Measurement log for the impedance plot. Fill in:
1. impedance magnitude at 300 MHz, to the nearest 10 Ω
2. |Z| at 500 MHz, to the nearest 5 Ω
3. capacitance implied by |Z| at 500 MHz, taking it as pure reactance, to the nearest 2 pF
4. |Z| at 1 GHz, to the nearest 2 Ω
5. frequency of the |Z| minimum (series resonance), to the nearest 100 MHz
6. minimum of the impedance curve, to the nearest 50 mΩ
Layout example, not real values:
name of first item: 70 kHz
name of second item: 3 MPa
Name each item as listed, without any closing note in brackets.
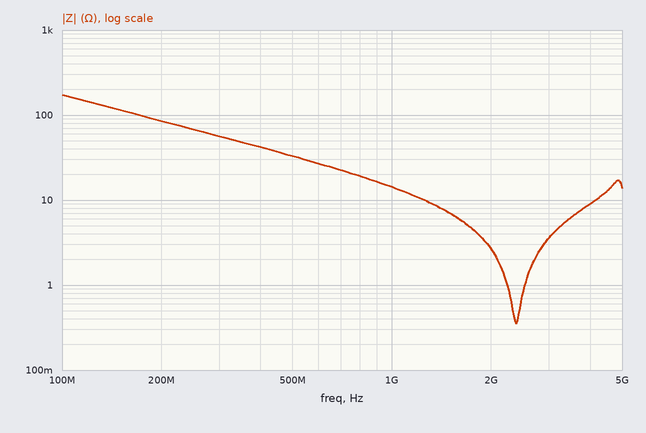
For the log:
impedance magnitude at 300 MHz, to the nearest 10 Ω: 60 Ω
|Z| at 500 MHz, to the nearest 5 Ω: 35 Ω
capacitance implied by |Z| at 500 MHz, taking it as pure reactance, to the nearest 2 pF: 10 pF
|Z| at 1 GHz, to the nearest 2 Ω: 14 Ω
frequency of the |Z| minimum (series resonance), to the nearest 100 MHz: 2.4 GHz
minimum of the impedance curve, to the nearest 50 mΩ: 350 mΩ
